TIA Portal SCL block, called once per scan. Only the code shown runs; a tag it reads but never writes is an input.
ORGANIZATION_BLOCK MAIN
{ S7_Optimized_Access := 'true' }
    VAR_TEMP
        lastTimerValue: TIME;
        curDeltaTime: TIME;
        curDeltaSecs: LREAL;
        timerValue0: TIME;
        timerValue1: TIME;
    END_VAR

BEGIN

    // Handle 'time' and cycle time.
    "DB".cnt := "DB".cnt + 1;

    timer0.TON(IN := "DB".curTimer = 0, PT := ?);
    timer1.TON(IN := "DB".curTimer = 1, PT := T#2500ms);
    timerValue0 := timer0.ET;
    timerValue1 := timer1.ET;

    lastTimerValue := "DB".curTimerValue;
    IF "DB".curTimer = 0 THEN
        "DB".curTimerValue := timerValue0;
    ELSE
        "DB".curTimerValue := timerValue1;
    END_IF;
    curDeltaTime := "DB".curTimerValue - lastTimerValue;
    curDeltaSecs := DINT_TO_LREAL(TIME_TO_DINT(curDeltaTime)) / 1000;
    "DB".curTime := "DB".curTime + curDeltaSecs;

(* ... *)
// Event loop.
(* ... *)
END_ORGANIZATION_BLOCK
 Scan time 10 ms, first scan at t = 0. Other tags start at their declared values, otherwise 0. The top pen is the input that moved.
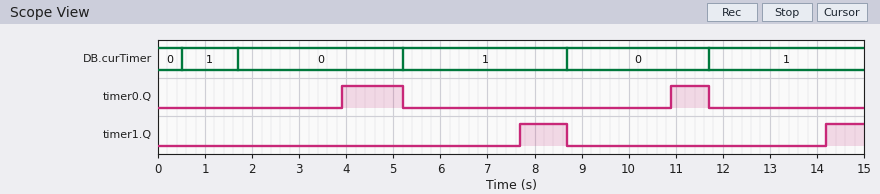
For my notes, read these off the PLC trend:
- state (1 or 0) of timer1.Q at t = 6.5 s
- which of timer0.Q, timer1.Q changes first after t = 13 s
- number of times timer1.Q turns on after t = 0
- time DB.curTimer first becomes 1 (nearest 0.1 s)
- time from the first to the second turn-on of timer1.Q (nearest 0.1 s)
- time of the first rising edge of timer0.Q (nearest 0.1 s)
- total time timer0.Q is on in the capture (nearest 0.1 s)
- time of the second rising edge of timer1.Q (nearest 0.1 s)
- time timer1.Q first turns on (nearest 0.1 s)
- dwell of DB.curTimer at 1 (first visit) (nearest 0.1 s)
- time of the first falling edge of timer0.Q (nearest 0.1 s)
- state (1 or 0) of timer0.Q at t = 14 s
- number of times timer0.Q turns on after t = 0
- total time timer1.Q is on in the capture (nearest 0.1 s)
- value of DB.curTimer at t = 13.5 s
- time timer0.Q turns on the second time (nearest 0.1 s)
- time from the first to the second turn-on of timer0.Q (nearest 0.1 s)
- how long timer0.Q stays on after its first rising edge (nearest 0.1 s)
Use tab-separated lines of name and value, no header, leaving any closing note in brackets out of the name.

state (1 or 0) of timer1.Q at t = 6.5 s	0
which of timer0.Q, timer1.Q changes first after t = 13 s	timer1.Q
number of times timer1.Q turns on after t = 0	2
time DB.curTimer first becomes 1	0.5 s
time from the first to the second turn-on of timer1.Q	6.5 s
time of the first rising edge of timer0.Q	3.9 s
total time timer0.Q is on in the capture	2.1 s
time of the second rising edge of timer1.Q	14.2 s
time timer1.Q first turns on	7.7 s
dwell of DB.curTimer at 1 (first visit)	1.2 s
time of the first falling edge of timer0.Q	5.2 s
state (1 or 0) of timer0.Q at t = 14 s	0
number of times timer0.Q turns on after t = 0	2
total time timer1.Q is on in the capture	1.8 s
value of DB.curTimer at t = 13.5 s	1
time timer0.Q turns on the second time	10.9 s
time from the first to the second turn-on of timer0.Q	7.0 s
how long timer0.Q stays on after its first rising edge	1.3 s
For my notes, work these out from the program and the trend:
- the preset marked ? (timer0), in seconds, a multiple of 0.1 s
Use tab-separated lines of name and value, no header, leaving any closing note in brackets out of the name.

the preset marked ? (timer0), in seconds, a multiple of 0.1 s	2.2 s
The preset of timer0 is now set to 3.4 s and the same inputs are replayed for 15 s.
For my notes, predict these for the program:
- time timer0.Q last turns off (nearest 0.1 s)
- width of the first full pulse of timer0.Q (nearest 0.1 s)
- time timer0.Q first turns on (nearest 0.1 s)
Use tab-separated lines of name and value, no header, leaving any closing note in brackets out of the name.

time timer0.Q last turns off	5.2 s
width of the first full pulse of timer0.Q	0.1 s
time timer0.Q first turns on	5.1 s
